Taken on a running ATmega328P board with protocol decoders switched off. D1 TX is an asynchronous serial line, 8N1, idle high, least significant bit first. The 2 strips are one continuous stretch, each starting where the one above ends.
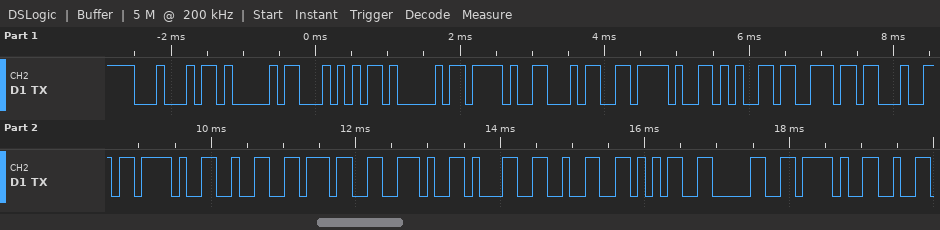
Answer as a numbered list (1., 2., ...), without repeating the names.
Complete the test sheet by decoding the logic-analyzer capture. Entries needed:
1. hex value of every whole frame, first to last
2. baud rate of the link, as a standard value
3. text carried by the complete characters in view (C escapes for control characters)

1. 44 41 54 41 2F 34 2F 65 6E 64 2F 32 37 2E 31 32 35 30 2F
2. 9600 baud
3. "DATA/4/end/27.1250/"
